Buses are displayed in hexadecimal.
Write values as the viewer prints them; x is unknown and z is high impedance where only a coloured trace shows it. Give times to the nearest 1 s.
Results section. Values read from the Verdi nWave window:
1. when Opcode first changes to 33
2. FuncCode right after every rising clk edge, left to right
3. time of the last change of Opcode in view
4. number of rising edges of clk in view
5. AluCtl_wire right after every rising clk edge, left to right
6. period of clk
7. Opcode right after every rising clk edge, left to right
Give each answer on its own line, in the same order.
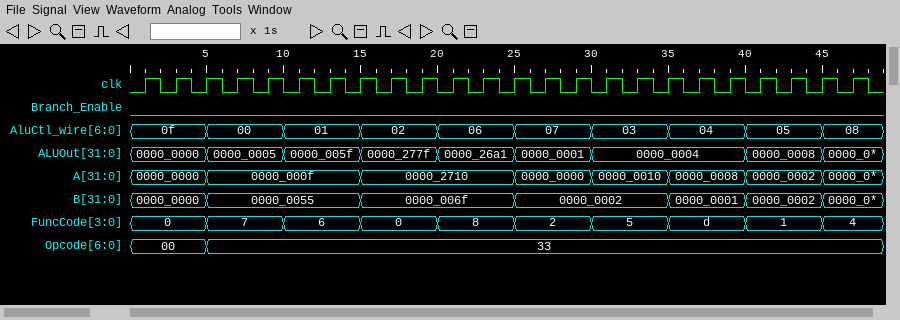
5 s
0, 0, 7, 7, 7, 6, 6, 0, 0, 0, 8, 8, 2, 2, 2, 5, 5, d, d, d, 1, 1, 4, 4
5 s
24
0f, 0f, 00, 00, 00, 01, 01, 02, 02, 02, 06, 06, 07, 07, 07, 03, 03, 04, 04, 04, 05, 05, 08, 08
2 s
00, 00, 33, 33, 33, 33, 33, 33, 33, 33, 33, 33, 33, 33, 33, 33, 33, 33, 33, 33, 33, 33, 33, 33
